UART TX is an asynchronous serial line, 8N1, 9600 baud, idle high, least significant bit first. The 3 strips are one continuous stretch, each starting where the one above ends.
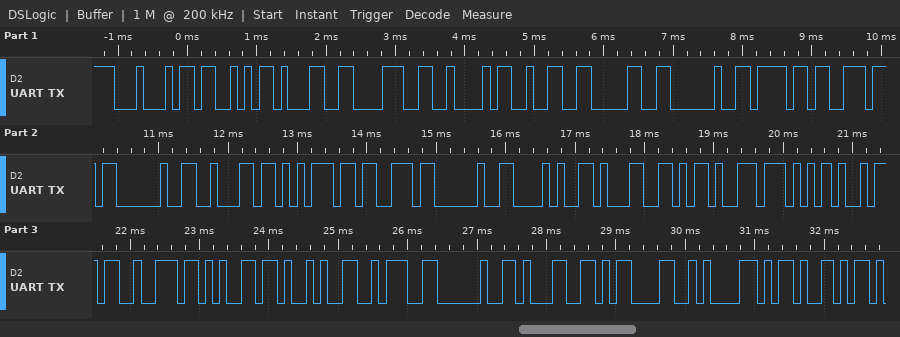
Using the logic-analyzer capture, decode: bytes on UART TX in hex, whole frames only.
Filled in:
44 53 31 38 42 32 30 20 6F 6E 20 62 75 73 20 28 31 2D 57 69 72 65 29 3A 20 31 0D 0A 2D
